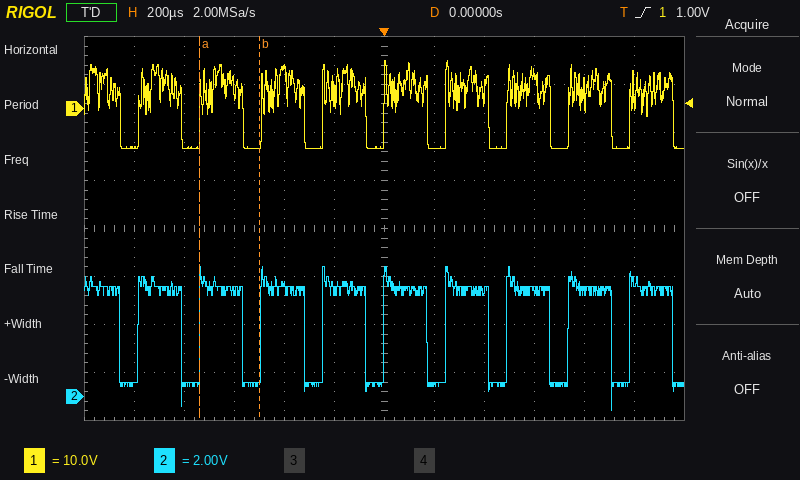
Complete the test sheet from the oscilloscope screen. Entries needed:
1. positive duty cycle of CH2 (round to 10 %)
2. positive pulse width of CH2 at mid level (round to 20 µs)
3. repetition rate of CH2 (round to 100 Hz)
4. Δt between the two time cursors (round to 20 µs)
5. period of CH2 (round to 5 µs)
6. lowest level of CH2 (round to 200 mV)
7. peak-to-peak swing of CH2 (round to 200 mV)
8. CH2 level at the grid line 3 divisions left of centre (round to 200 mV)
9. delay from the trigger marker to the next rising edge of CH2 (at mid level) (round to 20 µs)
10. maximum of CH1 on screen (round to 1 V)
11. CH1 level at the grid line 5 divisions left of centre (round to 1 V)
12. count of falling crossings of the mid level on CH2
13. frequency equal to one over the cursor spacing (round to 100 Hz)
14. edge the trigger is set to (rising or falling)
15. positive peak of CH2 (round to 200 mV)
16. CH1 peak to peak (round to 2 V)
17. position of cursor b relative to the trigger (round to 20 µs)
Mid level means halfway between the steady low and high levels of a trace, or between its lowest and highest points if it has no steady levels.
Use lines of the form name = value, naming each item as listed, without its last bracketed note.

positive duty cycle of CH2 = 70 %
positive pulse width of CH2 at mid level = 180 µs
repetition rate of CH2 = 4.1 kHz
Δt between the two time cursors = 240 µs
period of CH2 = 245 µs
lowest level of CH2 = -600 mV
peak-to-peak swing of CH2 = 6.0 V
CH2 level at the grid line 3 divisions left of centre = 4.4 V
delay from the trigger marker to the next rising edge of CH2 (at mid level) = 240 µs
maximum of CH1 on screen = 10 V
CH1 level at the grid line 5 divisions left of centre = -8 V
count of falling crossings of the mid level on CH2 = 10
frequency equal to one over the cursor spacing = 4.2 kHz
edge the trigger is set to = rising
positive peak of CH2 = 5.4 V
CH1 peak to peak = 18 V
position of cursor b relative to the trigger = -500 µs
